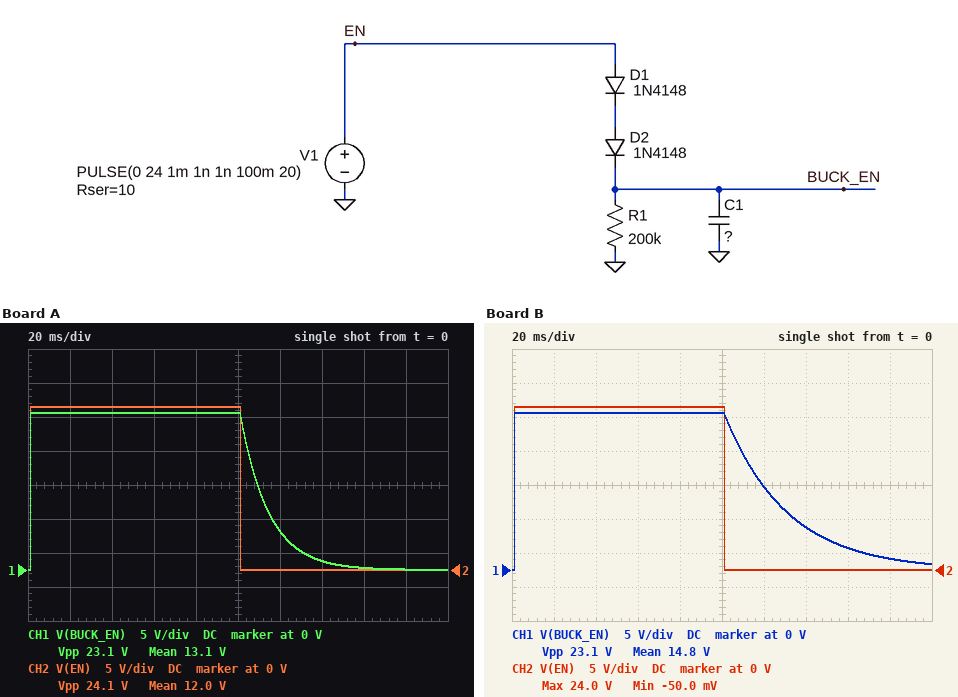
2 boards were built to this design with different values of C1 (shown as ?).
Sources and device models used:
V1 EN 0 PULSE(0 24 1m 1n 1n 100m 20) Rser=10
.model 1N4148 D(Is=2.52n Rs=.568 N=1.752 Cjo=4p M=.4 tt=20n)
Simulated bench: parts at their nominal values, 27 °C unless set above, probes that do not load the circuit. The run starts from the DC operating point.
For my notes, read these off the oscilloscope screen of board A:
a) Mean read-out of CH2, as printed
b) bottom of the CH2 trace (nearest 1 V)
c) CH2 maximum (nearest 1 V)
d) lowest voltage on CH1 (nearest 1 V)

12.0 V
0 V
24 V
0 V
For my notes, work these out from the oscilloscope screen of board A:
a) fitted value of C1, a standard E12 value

68 nF
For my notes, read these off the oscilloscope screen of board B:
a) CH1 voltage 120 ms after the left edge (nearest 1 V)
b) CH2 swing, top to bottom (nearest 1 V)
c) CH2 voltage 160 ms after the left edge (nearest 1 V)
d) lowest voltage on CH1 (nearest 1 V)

12 V
24 V
0 V
0 V
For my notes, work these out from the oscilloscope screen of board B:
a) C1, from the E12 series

150 nF
